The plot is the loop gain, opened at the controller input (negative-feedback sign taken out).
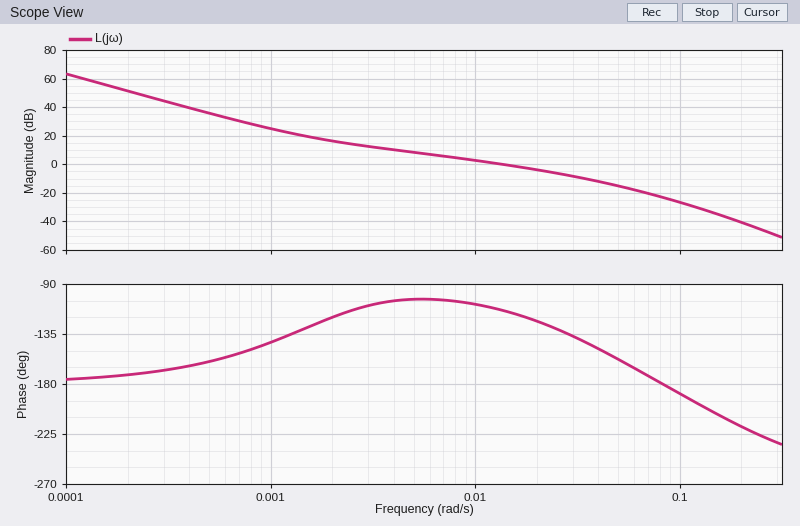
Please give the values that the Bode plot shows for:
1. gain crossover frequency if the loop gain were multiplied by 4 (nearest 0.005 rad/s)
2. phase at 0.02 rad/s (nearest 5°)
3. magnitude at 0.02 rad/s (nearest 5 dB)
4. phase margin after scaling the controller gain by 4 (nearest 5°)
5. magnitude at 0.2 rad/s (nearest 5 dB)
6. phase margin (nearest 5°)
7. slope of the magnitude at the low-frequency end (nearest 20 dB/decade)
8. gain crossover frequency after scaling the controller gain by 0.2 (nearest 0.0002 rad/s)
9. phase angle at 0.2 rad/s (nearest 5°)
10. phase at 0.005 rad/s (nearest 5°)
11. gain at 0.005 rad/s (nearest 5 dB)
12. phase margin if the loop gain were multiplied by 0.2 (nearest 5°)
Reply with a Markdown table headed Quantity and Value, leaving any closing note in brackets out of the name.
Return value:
| Quantity | Value |
|---|---|
| gain crossover frequency if the loop gain were multiplied by 4 | 0.040 rad/s |
| phase at 0.02 rad/s | -125° |
| magnitude at 0.02 rad/s | -5 dB |
| phase margin after scaling the controller gain by 4 | 30° |
| magnitude at 0.2 rad/s | -40 dB |
| phase margin | 65° |
| slope of the magnitude at the low-frequency end | -40 dB/decade |
| gain crossover frequency after scaling the controller gain by 0.2 | 0.0026 rad/s |
| phase angle at 0.2 rad/s | -220° |
| phase at 0.005 rad/s | -105° |
| gain at 0.005 rad/s | 10 dB |
| phase margin if the loop gain were multiplied by 0.2 | 65° |
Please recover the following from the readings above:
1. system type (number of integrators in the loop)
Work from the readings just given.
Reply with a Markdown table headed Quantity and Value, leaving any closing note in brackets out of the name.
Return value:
| Quantity | Value |
|---|---|
| system type | 2 |
